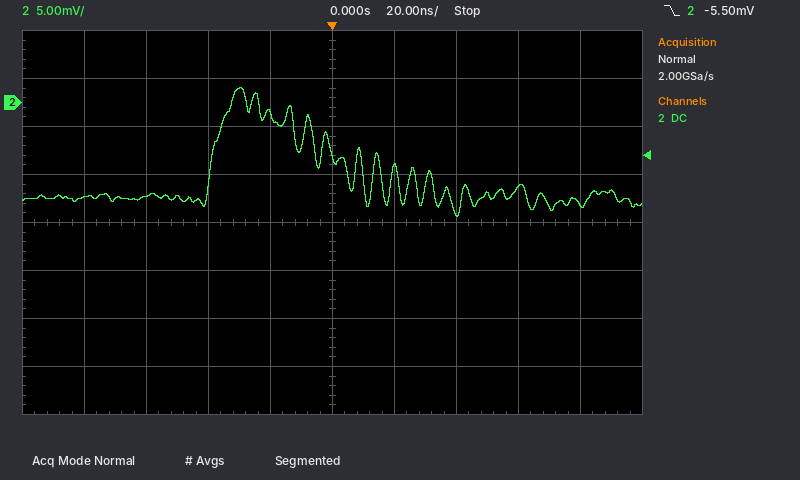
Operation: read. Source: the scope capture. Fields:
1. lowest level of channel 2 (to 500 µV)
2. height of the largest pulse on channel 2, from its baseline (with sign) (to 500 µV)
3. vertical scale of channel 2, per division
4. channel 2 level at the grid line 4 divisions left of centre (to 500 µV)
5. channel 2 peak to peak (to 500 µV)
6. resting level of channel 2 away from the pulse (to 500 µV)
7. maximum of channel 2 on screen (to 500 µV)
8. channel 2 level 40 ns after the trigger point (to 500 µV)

-12.0 mV
+11.5 mV
5 mV
-10.0 mV
13.5 mV
-10.0 mV
1.5 mV
-11.5 mV
